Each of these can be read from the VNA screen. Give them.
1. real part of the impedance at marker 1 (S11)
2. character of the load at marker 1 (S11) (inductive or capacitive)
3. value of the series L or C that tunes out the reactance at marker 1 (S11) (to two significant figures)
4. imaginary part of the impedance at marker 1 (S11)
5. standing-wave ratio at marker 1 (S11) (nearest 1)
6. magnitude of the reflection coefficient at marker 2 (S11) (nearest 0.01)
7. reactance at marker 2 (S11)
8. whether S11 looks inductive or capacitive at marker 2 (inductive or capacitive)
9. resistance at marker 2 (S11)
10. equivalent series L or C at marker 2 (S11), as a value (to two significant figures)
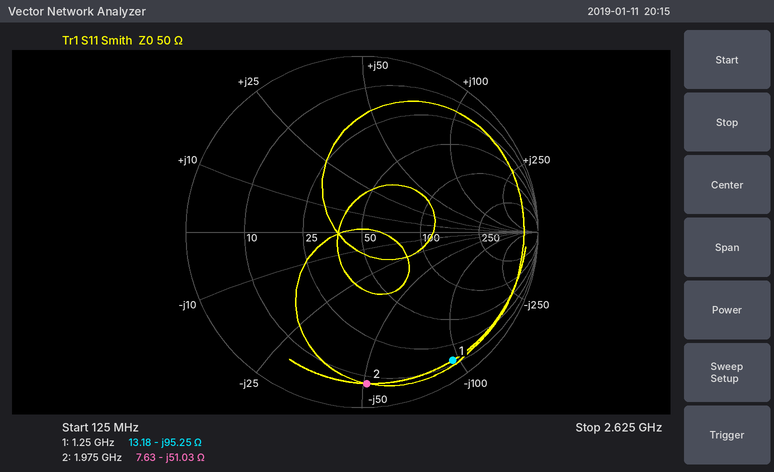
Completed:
13.18 Ω
capacitive
12 nH
-95.25 Ω
18
0.86
-51.03 Ω
capacitive
7.63 Ω
1.6 pF
